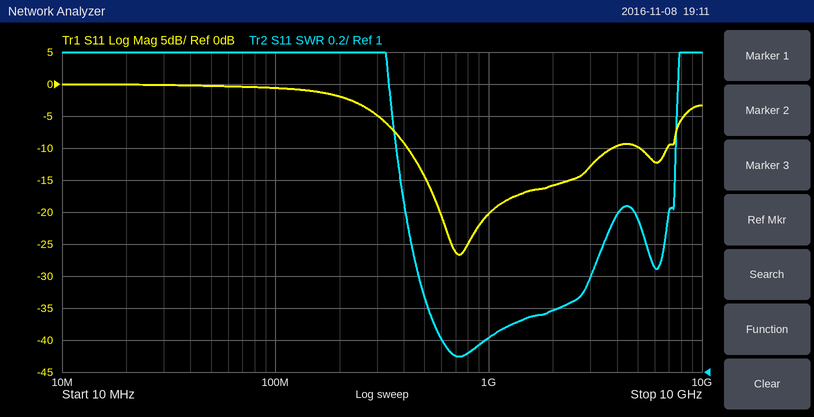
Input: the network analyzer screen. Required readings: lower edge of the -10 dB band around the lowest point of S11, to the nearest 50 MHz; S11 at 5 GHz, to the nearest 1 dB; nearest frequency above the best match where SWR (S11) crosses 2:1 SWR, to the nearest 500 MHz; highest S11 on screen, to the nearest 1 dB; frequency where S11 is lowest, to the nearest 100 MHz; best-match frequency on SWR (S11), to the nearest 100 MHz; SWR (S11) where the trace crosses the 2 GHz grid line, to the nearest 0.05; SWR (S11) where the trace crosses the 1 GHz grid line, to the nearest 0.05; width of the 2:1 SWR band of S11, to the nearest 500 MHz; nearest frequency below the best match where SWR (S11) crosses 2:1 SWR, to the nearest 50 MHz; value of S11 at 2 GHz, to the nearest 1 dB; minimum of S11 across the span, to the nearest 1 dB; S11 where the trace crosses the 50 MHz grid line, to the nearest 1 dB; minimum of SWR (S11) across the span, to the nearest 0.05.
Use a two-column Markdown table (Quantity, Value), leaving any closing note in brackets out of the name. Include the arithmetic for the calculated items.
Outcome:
| Quantity | Value |
|---|---|
| lower edge of the -10 dB band around the lowest point of S11, to the nearest 50 MHz | 400 MHz |
| S11 at 5 GHz, to the nearest 1 dB | -10 dB |
| nearest frequency above the best match where SWR (S11) crosses 2:1 SWR, to the nearest 500 MHz | 4.0 GHz |
| highest S11 on screen, to the nearest 1 dB | 0 dB |
| frequency where S11 is lowest, to the nearest 100 MHz | 700 MHz |
| best-match frequency on SWR (S11), to the nearest 100 MHz | 700 MHz |
| SWR (S11) where the trace crosses the 2 GHz grid line, to the nearest 0.05 | 1.40 |
| SWR (S11) where the trace crosses the 1 GHz grid line, to the nearest 0.05 | 1.20 |
| width of the 2:1 SWR band of S11, to the nearest 500 MHz | 4.0 GHz − 400 MHz = 3.60 GHz |
| nearest frequency below the best match where SWR (S11) crosses 2:1 SWR, to the nearest 50 MHz | 400 MHz |
| value of S11 at 2 GHz, to the nearest 1 dB | -16 dB |
| minimum of S11 across the span, to the nearest 1 dB | -27 dB |
| S11 where the trace crosses the 50 MHz grid line, to the nearest 1 dB | 0 dB |
| minimum of SWR (S11) across the span, to the nearest 0.05 | 1.10 |
